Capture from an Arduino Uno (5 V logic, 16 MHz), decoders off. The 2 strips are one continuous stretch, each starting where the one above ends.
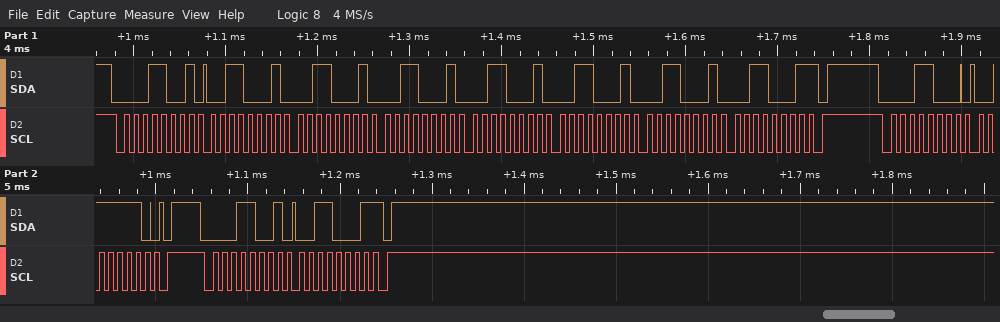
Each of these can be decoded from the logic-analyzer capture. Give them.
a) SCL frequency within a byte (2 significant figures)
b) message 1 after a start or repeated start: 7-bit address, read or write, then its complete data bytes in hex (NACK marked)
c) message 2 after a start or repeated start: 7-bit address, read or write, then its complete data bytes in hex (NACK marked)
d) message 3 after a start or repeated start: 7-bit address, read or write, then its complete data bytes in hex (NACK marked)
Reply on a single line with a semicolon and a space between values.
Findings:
100 kHz; 0x0C read: 31 31 31 31 31 31 31 NACK; 0x0C write: 3E; 0x0C read: 31 NACK
